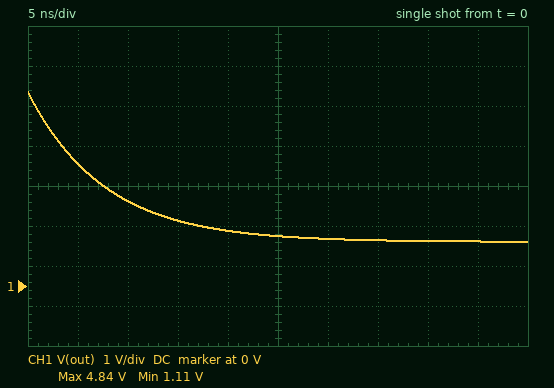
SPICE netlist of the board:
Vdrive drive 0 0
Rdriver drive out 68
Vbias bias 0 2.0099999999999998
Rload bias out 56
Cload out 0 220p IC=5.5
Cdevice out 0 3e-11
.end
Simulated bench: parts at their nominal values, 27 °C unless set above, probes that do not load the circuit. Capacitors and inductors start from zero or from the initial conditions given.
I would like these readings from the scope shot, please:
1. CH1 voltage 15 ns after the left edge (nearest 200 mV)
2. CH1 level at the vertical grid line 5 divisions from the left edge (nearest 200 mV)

1.6 V
1.2 V
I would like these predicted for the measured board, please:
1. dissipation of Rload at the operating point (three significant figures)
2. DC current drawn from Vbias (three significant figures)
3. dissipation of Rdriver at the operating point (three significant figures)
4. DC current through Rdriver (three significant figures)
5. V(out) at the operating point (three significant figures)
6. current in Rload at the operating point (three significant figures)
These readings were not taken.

14.7 mW
16.2 mA
17.9 mW
16.2 mA
1.10 V
16.2 mA
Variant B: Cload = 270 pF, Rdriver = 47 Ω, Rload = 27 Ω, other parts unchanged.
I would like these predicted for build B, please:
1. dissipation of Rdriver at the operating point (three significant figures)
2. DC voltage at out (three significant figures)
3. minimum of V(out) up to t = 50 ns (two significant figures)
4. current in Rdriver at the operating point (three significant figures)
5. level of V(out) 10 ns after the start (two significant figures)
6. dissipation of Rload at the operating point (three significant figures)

34.7 mW
1.28 V
1.3 V
27.2 mA
1.8 V
19.9 mW
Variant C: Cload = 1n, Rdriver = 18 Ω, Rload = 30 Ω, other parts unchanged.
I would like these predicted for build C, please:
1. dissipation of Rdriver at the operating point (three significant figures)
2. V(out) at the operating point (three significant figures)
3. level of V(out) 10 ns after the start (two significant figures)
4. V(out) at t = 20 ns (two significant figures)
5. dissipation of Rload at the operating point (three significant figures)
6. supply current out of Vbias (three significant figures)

31.6 mW
754 mV
2.7 V
1.6 V
52.6 mW
41.9 mA
